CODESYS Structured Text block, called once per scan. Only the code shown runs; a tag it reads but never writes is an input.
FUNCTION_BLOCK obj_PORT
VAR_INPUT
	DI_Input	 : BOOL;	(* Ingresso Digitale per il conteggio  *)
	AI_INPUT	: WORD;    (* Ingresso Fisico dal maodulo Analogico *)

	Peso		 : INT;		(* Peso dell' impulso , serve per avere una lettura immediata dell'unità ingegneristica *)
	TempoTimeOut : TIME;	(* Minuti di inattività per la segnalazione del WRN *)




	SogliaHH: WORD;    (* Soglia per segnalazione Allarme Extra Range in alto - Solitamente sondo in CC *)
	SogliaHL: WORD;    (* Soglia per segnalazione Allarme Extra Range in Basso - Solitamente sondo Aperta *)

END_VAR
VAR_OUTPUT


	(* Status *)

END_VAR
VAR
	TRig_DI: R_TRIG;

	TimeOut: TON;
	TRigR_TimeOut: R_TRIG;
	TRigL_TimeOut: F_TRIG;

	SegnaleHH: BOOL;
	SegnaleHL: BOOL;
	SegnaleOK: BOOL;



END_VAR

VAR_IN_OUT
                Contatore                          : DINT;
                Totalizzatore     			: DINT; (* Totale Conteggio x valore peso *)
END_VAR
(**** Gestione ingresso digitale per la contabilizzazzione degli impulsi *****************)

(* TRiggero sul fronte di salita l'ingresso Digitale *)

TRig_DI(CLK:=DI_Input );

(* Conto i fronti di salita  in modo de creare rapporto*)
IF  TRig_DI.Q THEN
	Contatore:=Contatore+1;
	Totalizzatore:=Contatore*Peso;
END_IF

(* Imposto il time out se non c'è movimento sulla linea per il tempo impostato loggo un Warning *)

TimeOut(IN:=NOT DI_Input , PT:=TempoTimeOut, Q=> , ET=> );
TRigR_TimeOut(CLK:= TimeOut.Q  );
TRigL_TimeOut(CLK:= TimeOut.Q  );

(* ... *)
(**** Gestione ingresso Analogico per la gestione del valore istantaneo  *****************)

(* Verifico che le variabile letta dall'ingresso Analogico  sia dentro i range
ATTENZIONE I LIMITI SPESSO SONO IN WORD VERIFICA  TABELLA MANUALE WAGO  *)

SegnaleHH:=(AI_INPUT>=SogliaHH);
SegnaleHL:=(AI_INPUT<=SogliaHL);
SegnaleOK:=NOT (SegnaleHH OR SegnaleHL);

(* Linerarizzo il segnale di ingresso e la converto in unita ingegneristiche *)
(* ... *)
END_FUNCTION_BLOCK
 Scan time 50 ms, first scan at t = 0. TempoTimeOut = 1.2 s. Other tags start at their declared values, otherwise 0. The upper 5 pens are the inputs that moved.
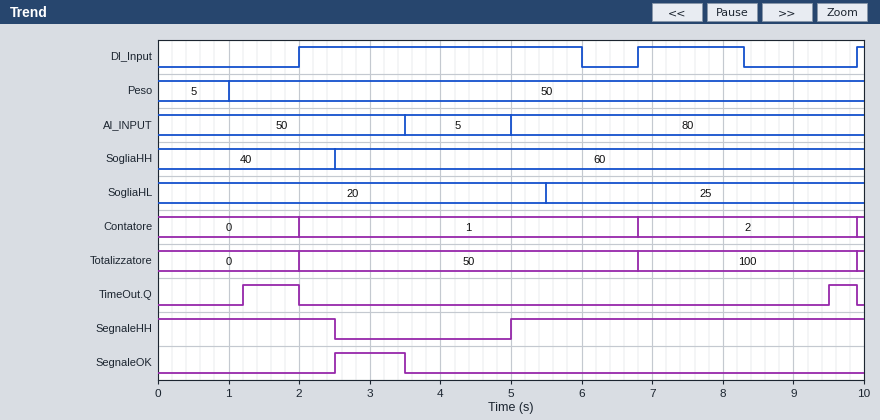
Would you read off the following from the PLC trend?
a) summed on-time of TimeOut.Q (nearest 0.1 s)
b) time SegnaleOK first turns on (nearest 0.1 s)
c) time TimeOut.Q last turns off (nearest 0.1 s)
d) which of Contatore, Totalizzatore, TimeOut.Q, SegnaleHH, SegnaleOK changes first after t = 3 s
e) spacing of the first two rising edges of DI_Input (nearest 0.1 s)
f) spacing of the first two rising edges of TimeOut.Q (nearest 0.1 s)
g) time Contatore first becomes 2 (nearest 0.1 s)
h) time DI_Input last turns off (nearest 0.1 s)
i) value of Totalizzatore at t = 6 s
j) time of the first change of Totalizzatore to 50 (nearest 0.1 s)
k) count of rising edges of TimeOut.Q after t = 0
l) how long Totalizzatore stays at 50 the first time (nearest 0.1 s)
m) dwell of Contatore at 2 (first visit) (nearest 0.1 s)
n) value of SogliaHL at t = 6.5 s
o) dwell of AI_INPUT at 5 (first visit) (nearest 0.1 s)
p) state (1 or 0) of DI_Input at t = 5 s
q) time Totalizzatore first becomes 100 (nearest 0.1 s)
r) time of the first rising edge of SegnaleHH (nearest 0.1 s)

1.2 s
2.5 s
9.9 s
SegnaleOK
4.8 s
8.3 s
6.8 s
8.3 s
50
2.0 s
2
4.8 s
3.1 s
25
1.5 s
1
6.8 s
5.0 s
